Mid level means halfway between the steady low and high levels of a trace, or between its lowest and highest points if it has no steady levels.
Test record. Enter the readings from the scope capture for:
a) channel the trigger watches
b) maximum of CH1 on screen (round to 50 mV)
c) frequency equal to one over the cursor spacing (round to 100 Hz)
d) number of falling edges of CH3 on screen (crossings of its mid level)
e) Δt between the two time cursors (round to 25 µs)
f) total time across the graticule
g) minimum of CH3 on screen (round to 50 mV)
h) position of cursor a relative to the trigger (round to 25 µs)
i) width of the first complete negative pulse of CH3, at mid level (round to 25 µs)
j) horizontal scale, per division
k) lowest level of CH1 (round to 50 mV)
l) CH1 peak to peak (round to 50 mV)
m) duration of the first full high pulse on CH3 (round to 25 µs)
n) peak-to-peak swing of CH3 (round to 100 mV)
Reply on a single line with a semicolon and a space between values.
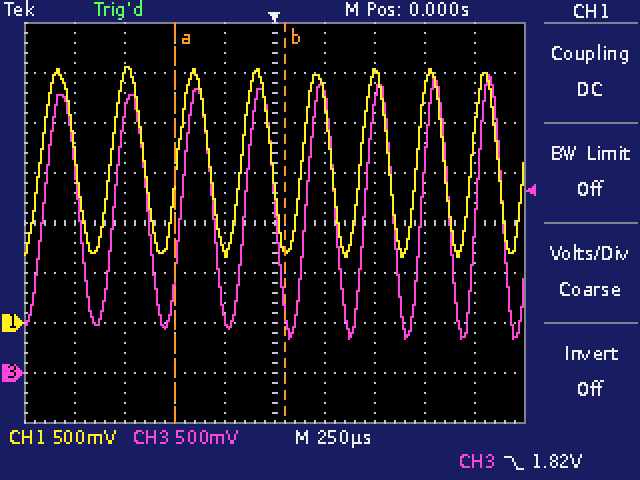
CH3; 2.55 V; 1.8 kHz; 8; 550 µs; 2.5 ms; 350 mV; -500 µs; 175 µs; 250 µs; 650 mV; 1.90 V; 175 µs; 2.60 V
